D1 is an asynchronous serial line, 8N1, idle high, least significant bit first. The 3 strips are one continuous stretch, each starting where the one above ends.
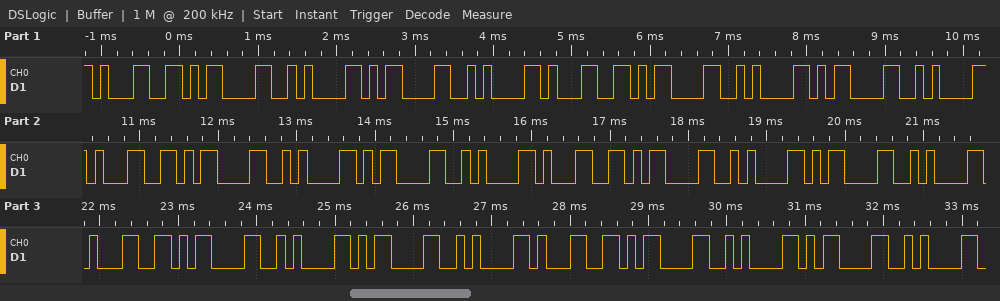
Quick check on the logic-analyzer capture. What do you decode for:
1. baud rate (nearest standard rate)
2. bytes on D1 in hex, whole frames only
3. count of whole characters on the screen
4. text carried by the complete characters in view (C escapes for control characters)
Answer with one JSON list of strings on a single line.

["9600 baud", "31 0D 0A 0D 0A 31 0D 0A 0D 0A 31 0D 0A 0D 0A 31 0D 0A 0D 0A 31 0D 0A 0D 0A 31 0D 0A 0D 0A", "30", "\"1\\r\\n\\r\\n1\\r\\n\\r\\n1\\r\\n\\r\\n1\\r\\n\\r\\n1\\r\\n\\r\\n1\\r\\n\\r\\n\""]
